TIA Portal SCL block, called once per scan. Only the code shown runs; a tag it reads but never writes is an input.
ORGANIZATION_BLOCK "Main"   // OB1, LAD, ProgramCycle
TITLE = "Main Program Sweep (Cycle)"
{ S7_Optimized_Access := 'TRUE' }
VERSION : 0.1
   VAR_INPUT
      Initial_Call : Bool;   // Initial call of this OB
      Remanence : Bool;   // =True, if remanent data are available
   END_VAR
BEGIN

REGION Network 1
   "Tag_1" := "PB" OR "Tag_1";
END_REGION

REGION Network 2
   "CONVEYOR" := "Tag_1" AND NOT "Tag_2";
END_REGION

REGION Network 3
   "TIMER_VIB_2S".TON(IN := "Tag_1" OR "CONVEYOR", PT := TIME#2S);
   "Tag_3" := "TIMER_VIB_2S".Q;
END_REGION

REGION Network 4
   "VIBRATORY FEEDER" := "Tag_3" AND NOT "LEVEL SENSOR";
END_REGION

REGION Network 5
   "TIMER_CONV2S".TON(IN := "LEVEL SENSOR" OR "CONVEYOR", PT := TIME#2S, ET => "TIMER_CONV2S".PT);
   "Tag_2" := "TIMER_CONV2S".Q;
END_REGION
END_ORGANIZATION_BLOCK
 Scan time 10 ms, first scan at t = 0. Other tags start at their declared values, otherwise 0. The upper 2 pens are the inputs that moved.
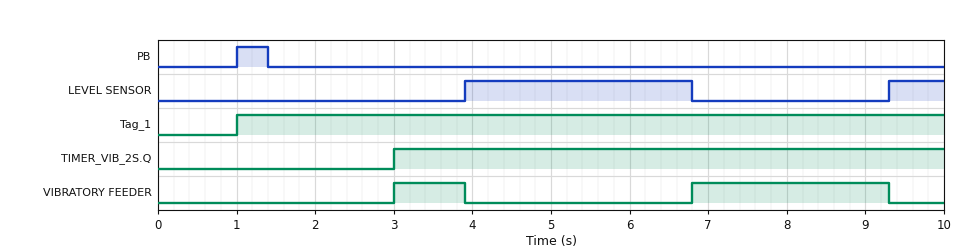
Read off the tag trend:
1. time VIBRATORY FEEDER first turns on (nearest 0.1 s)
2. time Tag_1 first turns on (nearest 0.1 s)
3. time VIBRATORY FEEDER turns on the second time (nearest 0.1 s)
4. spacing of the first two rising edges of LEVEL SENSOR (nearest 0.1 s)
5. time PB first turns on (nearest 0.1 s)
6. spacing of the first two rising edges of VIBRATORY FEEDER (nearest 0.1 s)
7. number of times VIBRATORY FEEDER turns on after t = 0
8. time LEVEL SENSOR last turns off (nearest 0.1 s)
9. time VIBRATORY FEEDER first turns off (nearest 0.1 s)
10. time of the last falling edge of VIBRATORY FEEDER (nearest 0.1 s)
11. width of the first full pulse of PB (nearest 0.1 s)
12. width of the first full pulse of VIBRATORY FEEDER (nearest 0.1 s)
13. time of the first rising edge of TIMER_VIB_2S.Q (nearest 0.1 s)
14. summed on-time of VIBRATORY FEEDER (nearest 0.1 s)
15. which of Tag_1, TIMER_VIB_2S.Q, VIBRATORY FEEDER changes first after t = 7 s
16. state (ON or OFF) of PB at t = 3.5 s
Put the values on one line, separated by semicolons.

3.0 s; 1.0 s; 6.8 s; 5.4 s; 1.0 s; 3.8 s; 2; 6.8 s; 3.9 s; 9.3 s; 0.4 s; 0.9 s; 3.0 s; 3.4 s; VIBRATORY FEEDER; OFF
